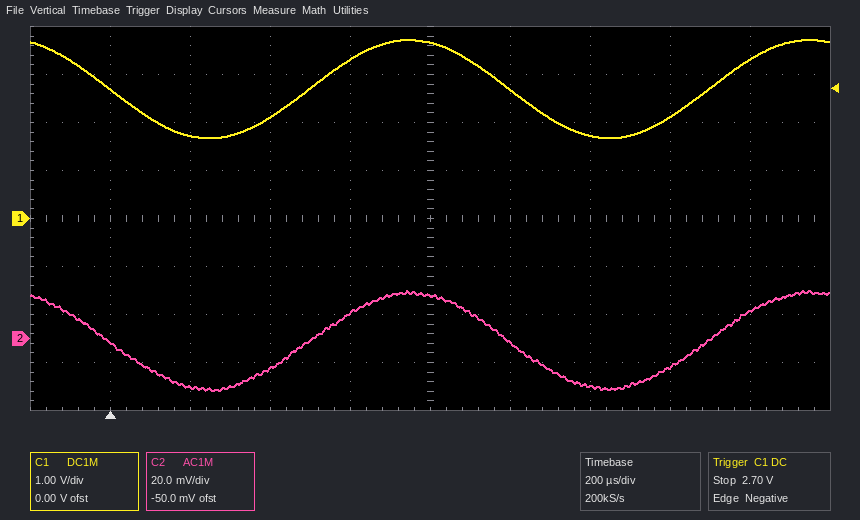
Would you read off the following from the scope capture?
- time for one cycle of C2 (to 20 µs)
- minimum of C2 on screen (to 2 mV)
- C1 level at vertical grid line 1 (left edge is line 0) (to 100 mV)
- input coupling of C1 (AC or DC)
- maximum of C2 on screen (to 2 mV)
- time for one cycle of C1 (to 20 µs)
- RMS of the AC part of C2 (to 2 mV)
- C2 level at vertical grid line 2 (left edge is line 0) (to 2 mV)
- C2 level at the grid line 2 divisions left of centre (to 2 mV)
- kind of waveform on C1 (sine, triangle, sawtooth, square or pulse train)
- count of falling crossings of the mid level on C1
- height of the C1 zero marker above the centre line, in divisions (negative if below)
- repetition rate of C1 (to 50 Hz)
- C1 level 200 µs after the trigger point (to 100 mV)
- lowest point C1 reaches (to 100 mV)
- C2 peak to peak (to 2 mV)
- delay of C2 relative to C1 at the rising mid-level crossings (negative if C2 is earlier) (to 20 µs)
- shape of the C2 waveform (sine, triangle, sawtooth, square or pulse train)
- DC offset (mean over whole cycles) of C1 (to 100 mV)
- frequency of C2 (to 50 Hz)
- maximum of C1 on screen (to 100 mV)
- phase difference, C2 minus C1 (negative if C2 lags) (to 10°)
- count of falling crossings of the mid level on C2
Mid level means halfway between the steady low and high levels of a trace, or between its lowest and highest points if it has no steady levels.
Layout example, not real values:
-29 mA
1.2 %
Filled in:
1.00 ms
-22 mV
2.7 V
DC
20 mV
1.00 ms
14 mV
-20 mV
-12 mV
sine
2
0.0 div
1.00 kHz
1.7 V
1.7 V
42 mV
0 µs
sine
2.7 V
1.00 kHz
3.7 V
0°
2
